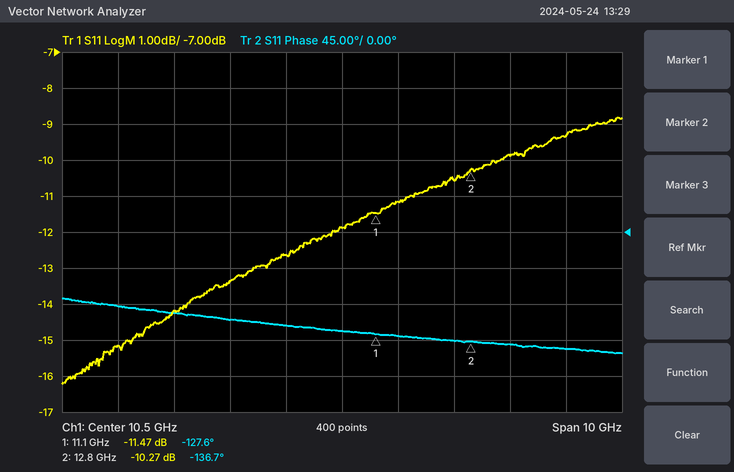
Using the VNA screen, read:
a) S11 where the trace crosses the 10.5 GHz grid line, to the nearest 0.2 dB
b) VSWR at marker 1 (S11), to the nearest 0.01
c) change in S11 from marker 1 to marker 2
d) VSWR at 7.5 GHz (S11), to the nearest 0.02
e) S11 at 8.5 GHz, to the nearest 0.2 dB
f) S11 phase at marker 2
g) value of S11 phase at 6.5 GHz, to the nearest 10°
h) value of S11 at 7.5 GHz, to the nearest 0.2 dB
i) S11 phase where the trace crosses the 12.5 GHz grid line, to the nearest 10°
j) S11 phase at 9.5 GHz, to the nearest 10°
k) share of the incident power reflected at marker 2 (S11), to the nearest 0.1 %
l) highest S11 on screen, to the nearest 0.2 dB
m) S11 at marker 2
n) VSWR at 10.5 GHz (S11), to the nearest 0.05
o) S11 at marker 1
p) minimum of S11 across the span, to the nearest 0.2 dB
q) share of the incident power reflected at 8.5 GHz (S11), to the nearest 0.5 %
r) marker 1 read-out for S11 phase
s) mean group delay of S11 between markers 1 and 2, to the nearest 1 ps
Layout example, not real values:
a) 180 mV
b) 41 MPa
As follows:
a) -11.8 dB
b) 1.73
c) 1.20 dB
d) 1.48
e) -13.4 dB
f) -136.7°
g) -90°
h) -14.2 dB
i) -140°
j) -120°
k) 9.4 %
l) -8.8 dB
m) -10.27 dB
n) 1.70
o) -11.47 dB
p) -16.2 dB
q) 4.5 %
r) -127.6°
s) 15 ps
